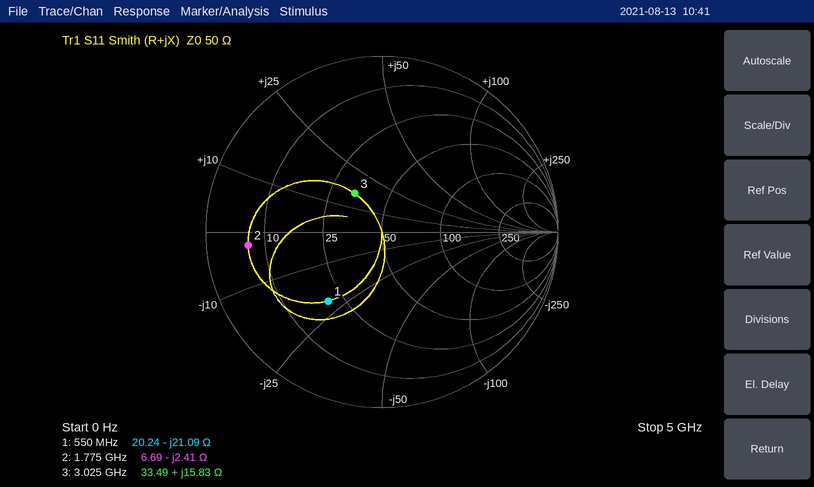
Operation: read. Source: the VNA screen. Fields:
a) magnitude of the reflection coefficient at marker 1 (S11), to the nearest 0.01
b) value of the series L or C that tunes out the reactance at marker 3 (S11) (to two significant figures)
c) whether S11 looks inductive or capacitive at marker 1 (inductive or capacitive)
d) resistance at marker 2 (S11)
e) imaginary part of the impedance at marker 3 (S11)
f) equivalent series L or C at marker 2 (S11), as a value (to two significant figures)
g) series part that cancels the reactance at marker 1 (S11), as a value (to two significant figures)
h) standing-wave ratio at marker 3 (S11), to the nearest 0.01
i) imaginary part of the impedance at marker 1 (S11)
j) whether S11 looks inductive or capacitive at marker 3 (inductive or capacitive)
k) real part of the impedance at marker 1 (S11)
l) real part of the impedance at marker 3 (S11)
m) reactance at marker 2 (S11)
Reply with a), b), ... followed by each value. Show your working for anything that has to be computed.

a) 0.50
b) C = 1/(2π × 3.025 GHz × 15.83 Ω) ≈ 3.3 pF
c) capacitive
d) 6.69 Ω
e) +15.83 Ω
f) C = 1/(2π × 1.775 GHz × 2.41 Ω) ≈ 37 pF
g) L = 21.09 Ω/(2π × 550 MHz) ≈ 6.1 nH
h) 1.74
i) -21.09 Ω
j) inductive
k) 20.24 Ω
l) 33.49 Ω
m) -2.41 Ω
